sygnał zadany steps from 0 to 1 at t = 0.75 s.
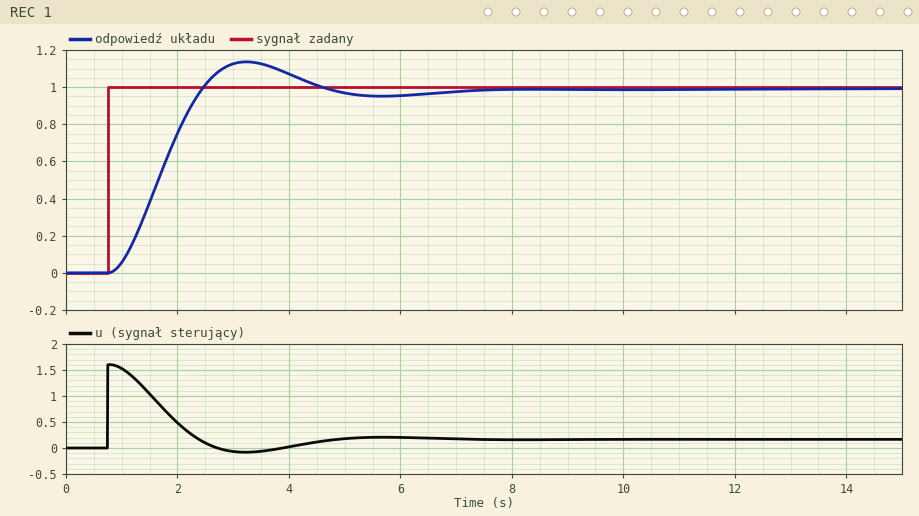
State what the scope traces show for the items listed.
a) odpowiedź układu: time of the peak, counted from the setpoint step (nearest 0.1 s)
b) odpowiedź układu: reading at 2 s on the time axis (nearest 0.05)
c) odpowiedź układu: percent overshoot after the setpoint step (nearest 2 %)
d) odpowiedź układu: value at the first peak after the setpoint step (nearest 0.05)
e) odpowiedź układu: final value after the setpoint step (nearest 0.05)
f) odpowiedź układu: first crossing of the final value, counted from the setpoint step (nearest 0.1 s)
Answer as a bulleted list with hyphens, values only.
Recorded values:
- 2.5 s
- 0.75
- 14 %
- 1.15
- 1.00
- 1.7 s
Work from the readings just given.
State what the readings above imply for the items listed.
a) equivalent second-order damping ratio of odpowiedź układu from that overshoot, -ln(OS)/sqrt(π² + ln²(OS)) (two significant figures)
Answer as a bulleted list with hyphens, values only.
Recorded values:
- 0.53
